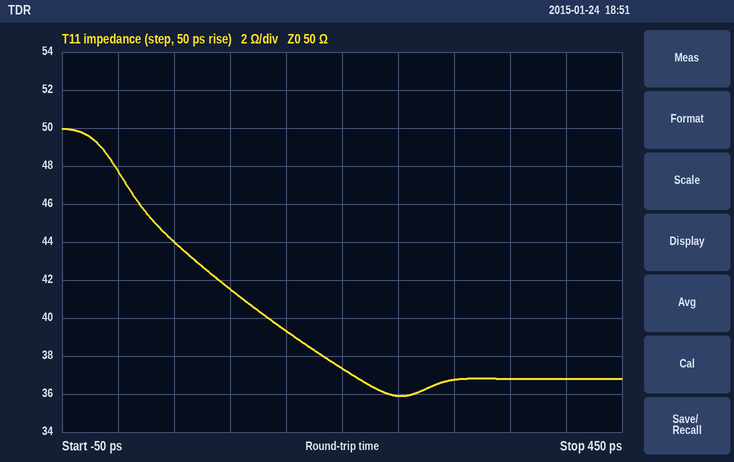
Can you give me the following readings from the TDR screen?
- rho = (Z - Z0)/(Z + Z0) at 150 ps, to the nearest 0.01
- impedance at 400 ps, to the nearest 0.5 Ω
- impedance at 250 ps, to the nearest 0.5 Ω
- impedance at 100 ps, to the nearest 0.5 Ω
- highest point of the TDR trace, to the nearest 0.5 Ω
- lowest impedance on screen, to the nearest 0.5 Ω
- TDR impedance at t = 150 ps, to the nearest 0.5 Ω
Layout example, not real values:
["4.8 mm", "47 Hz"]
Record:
["-0.12", "37.0 Ω", "36.0 Ω", "41.5 Ω", "50.0 Ω", "36.0 Ω", "39.5 Ω"]
